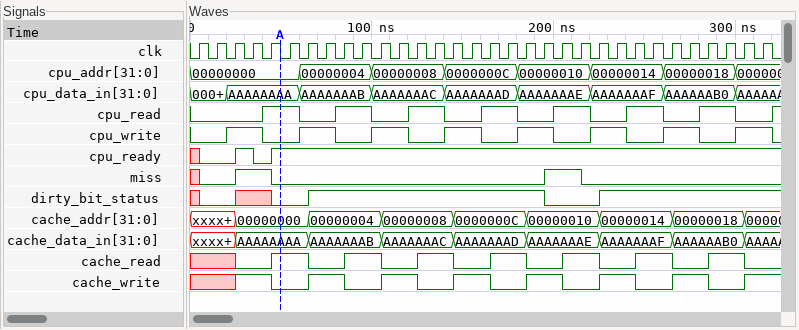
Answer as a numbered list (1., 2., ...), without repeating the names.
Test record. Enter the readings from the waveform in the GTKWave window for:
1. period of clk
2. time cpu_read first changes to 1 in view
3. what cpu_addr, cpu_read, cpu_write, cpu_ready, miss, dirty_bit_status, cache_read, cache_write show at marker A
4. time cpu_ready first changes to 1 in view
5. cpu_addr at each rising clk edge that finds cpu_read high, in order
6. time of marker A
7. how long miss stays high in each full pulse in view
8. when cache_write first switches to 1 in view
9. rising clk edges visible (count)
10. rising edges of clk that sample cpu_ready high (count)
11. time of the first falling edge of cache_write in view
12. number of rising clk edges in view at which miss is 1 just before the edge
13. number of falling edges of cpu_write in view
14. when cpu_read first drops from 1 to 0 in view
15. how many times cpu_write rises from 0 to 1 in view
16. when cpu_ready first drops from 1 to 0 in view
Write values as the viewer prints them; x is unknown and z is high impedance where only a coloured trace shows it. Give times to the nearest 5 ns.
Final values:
1. 10 ns
2. 40 ns
3. cpu_addr=00000000, cpu_read=1, cpu_write=0, cpu_ready=1, miss=0, dirty_bit_status=0, cache_read=1, cache_write=0
4. 25 ns
5. 00000000, 00000000, 00000004, 00000004, 00000008, 00000008, 0000000C, 0000000C, 00000010, 00000010, 00000014, 00000014, 00000018, 00000018
6. 50 ns
7. 20 ns, 20 ns
8. 25 ns
9. 32
10. 28
11. 45 ns
12. 4
13. 8
14. 60 ns
15. 8
16. 35 ns
